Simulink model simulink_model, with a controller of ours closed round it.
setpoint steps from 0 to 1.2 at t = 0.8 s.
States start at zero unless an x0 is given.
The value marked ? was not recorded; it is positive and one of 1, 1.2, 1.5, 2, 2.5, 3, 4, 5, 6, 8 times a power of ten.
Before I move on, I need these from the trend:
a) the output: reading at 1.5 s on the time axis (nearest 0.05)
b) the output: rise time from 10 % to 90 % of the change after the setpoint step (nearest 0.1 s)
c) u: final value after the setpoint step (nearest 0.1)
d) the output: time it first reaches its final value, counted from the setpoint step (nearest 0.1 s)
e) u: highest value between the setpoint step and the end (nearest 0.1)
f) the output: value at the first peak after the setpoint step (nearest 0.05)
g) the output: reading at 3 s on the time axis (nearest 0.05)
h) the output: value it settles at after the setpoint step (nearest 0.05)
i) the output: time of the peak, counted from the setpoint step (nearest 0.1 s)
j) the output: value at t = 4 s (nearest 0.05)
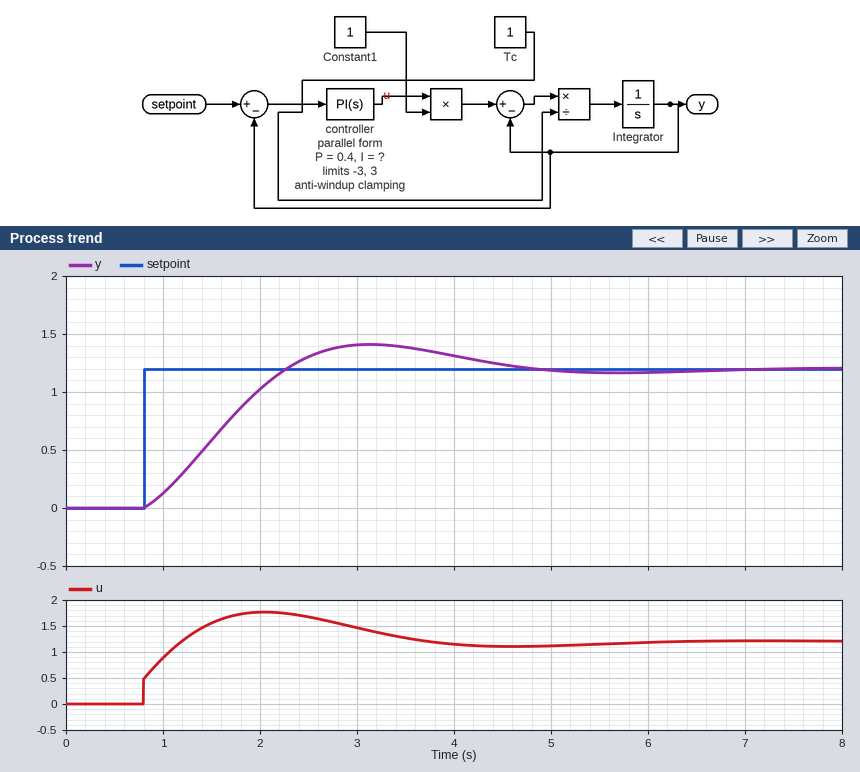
0.60
1.1 s
1.2
1.5 s
1.8
1.40
1.40
1.20
2.3 s
1.30
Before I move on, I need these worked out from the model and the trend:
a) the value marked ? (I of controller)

2
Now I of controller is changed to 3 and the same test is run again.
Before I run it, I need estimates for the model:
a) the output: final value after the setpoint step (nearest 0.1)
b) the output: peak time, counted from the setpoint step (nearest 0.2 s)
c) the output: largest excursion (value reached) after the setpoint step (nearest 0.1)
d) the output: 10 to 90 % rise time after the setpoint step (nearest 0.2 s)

1.2
1.8 s
1.5
0.8 s
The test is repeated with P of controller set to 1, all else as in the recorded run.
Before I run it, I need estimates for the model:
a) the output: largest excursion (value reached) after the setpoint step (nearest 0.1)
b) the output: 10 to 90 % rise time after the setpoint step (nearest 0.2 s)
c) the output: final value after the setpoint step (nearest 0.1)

1.3
1.2 s
1.2
